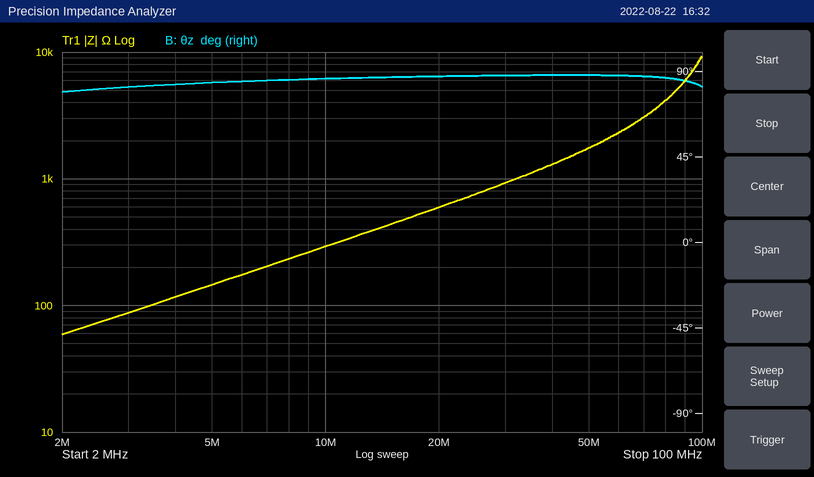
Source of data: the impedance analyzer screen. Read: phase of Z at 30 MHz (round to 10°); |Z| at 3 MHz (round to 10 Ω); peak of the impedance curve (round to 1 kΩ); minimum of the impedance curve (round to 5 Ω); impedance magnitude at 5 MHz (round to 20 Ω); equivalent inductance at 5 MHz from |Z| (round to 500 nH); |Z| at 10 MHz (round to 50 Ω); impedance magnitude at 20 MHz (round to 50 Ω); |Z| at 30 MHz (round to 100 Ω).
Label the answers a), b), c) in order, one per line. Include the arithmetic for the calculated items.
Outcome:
a) 90°
b) 90 Ω
c) 9 kΩ
d) 60 Ω
e) 140 Ω
f) L = 140 Ω/(2π × 5 MHz) ≈ 4.5 µH
g) 300 Ω
h) 600 Ω
i) 900 Ω
